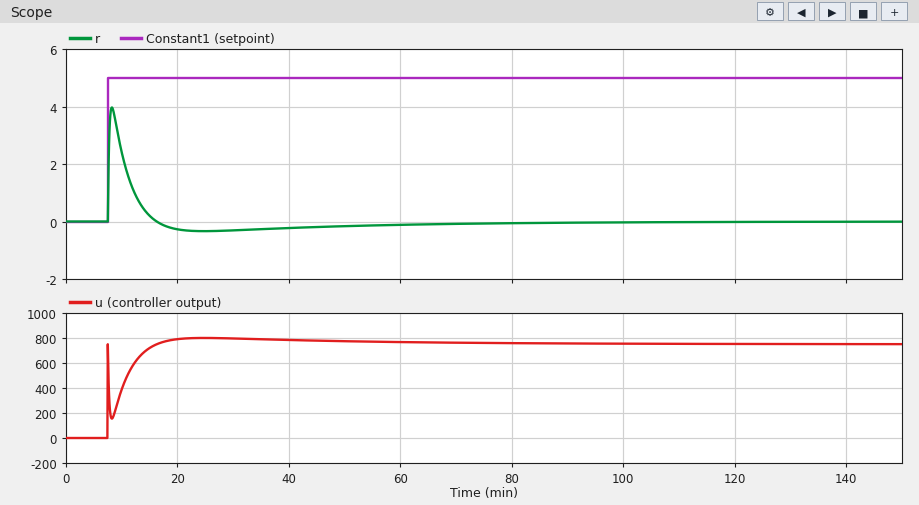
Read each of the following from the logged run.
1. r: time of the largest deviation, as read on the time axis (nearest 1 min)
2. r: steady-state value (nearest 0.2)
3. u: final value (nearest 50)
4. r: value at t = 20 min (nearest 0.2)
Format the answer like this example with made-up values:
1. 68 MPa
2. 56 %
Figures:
1. 8 min
2. 0.0
3. 750
4. -0.2
